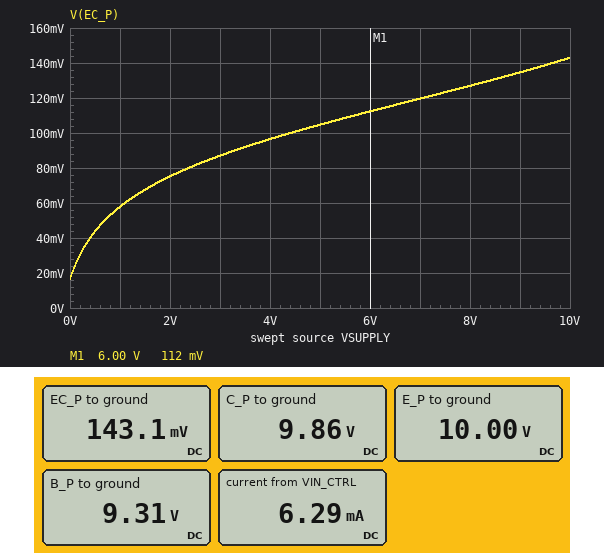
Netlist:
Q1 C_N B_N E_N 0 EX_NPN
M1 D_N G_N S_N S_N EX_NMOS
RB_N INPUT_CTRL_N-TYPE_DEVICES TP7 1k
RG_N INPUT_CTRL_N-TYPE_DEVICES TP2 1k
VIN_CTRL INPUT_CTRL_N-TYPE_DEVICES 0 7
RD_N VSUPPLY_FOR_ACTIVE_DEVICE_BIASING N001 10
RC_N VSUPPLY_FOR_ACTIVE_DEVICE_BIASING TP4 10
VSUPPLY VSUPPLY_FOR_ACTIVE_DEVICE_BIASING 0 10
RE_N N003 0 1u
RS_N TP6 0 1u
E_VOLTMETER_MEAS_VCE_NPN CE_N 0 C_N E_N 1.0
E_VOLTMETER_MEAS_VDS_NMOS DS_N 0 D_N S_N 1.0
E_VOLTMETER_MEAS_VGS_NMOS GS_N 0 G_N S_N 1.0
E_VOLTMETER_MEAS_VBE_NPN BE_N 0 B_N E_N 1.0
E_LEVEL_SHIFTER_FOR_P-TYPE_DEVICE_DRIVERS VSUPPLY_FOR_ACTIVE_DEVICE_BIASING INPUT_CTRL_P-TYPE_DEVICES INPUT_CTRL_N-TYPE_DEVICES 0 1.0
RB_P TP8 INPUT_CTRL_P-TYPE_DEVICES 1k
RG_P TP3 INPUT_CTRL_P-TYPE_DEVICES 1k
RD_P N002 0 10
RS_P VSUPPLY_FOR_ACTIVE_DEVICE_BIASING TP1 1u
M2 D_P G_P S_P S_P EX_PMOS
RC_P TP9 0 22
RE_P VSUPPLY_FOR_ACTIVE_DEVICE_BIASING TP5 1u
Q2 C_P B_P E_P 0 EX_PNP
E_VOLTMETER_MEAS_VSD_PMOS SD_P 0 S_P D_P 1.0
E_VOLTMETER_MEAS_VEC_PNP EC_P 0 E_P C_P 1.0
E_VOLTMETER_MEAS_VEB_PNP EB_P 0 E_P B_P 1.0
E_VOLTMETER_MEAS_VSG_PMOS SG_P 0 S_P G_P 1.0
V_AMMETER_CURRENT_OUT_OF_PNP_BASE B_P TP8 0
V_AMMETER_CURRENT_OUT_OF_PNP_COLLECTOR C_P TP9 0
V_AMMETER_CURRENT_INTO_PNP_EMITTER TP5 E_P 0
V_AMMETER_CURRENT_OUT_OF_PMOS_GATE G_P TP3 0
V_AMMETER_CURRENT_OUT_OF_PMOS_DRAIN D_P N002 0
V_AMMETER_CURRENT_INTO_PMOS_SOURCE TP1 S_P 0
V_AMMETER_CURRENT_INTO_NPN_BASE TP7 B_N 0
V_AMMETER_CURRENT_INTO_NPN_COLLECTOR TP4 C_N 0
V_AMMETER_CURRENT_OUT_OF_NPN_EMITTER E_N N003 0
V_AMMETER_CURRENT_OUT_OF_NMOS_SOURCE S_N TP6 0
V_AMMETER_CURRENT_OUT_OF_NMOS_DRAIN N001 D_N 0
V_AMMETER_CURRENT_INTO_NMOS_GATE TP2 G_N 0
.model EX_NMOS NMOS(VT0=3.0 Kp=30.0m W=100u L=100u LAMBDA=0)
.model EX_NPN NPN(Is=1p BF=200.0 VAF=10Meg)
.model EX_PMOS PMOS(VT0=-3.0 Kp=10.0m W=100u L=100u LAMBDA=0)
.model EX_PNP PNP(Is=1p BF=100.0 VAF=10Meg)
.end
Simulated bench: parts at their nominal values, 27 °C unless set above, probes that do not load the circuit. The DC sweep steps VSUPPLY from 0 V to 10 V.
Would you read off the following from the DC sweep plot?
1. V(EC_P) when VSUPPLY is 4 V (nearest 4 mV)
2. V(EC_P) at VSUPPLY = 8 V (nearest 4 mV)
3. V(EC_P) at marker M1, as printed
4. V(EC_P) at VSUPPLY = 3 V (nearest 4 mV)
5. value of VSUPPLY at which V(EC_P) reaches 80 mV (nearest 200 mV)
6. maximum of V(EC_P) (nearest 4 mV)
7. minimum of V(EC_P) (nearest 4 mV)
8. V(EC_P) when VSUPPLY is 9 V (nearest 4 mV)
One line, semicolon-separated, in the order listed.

96 mV; 128 mV; 112 mV; 88 mV; 2.4 V; 144 mV; 16 mV; 136 mV
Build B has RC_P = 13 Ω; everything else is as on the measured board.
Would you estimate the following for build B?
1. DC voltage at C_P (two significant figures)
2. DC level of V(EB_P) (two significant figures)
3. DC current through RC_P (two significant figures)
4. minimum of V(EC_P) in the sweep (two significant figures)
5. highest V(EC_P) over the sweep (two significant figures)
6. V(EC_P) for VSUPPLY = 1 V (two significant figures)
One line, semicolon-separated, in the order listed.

8.2 V; 700 mV; 630 mA; 15 mV; 1.8 V; 70 mV
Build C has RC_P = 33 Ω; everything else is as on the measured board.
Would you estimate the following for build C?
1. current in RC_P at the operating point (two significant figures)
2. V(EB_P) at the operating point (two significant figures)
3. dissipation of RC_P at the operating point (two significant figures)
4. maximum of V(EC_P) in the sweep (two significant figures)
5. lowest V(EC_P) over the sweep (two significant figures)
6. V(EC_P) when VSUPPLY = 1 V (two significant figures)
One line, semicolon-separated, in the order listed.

300 mA; 680 mV; 3.0 W; 120 mV; 17 mV; 50 mV
